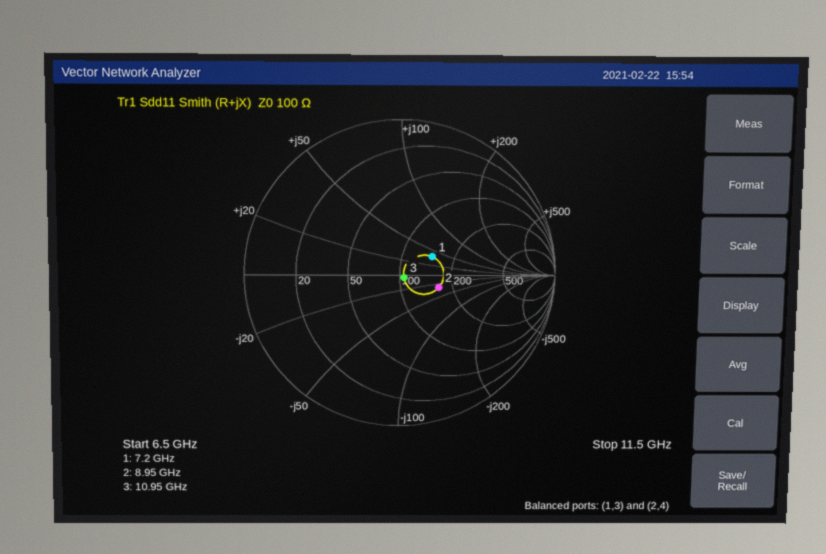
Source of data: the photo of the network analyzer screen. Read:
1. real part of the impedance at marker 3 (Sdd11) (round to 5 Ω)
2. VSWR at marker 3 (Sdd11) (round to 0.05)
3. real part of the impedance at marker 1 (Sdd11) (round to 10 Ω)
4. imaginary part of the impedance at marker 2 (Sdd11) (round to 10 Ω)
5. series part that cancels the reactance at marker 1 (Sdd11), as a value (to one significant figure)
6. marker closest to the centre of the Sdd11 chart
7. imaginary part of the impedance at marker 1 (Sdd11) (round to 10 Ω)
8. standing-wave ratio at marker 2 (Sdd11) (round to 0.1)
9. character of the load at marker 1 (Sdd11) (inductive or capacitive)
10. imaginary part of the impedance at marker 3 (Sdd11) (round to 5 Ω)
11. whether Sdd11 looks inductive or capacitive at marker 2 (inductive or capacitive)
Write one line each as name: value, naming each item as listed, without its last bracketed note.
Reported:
real part of the impedance at marker 3 (Sdd11): 105 Ω
VSWR at marker 3 (Sdd11): 1.05
real part of the impedance at marker 1 (Sdd11): 150 Ω
imaginary part of the impedance at marker 2 (Sdd11): -30 Ω
series part that cancels the reactance at marker 1 (Sdd11), as a value: 600 fF
marker closest to the centre of the Sdd11 chart: marker 3
imaginary part of the impedance at marker 1 (Sdd11): +40 Ω
standing-wave ratio at marker 2 (Sdd11): 1.7
character of the load at marker 1 (Sdd11): inductive
imaginary part of the impedance at marker 3 (Sdd11): -5 Ω
whether Sdd11 looks inductive or capacitive at marker 2: capacitive
